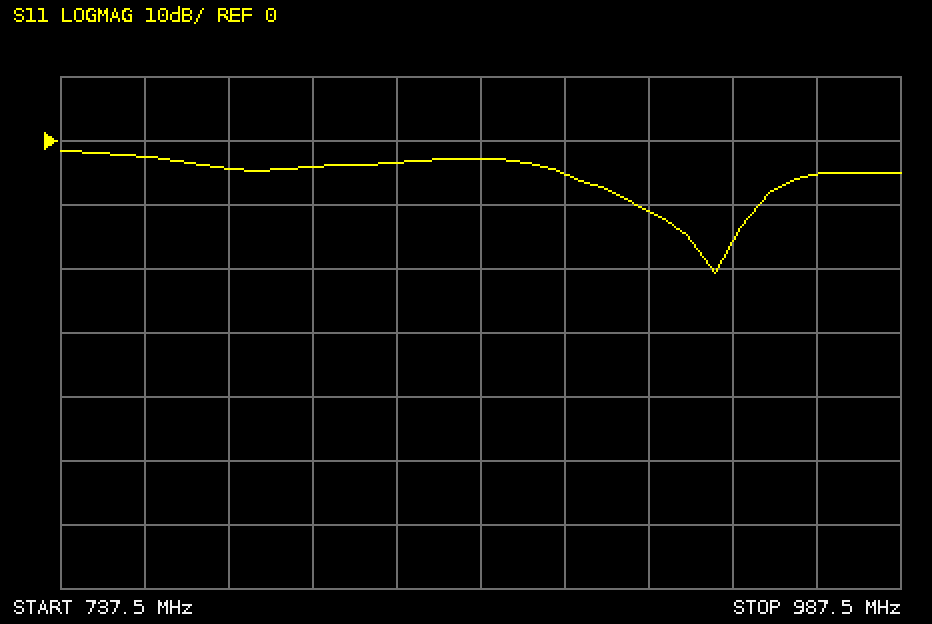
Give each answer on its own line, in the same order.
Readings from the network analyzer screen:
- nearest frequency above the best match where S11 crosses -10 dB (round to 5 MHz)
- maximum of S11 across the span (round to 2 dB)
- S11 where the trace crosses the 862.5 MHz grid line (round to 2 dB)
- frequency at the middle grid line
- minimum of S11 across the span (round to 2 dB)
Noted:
945 MHz
-2 dB
-2 dB
862.5 MHz
-20 dB
